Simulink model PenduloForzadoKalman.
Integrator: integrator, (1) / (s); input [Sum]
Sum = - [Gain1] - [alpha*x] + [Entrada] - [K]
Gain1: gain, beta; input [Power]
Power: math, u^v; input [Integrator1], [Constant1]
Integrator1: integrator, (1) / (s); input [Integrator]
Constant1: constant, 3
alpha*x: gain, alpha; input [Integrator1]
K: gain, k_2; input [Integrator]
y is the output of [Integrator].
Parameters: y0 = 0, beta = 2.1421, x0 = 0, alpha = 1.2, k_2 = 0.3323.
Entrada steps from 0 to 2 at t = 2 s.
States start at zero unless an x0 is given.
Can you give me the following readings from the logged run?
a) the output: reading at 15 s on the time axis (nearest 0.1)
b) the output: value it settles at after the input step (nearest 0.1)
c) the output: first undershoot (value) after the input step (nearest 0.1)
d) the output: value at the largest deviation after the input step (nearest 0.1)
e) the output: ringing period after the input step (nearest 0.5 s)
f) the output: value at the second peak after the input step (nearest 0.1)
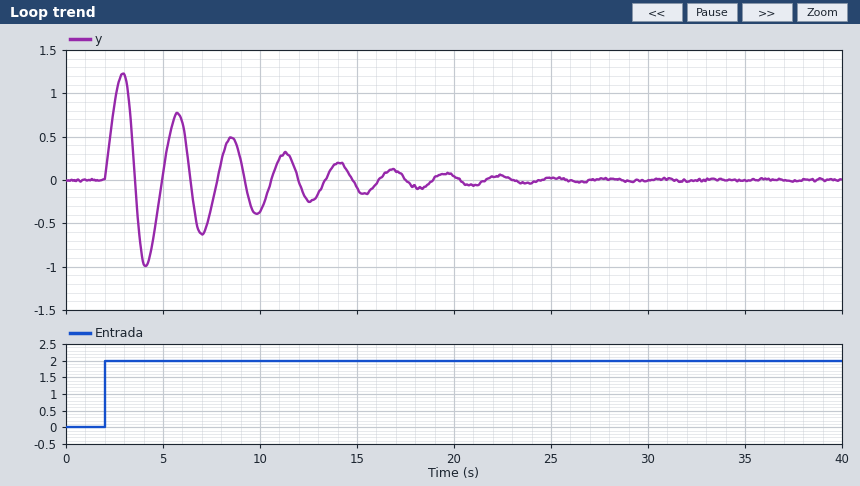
-0.1
0.0
-1.0
1.2
3.0 s
0.8
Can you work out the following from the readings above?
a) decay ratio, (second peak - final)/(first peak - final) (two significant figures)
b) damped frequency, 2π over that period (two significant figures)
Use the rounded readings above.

0.67
2.1 rad/s
